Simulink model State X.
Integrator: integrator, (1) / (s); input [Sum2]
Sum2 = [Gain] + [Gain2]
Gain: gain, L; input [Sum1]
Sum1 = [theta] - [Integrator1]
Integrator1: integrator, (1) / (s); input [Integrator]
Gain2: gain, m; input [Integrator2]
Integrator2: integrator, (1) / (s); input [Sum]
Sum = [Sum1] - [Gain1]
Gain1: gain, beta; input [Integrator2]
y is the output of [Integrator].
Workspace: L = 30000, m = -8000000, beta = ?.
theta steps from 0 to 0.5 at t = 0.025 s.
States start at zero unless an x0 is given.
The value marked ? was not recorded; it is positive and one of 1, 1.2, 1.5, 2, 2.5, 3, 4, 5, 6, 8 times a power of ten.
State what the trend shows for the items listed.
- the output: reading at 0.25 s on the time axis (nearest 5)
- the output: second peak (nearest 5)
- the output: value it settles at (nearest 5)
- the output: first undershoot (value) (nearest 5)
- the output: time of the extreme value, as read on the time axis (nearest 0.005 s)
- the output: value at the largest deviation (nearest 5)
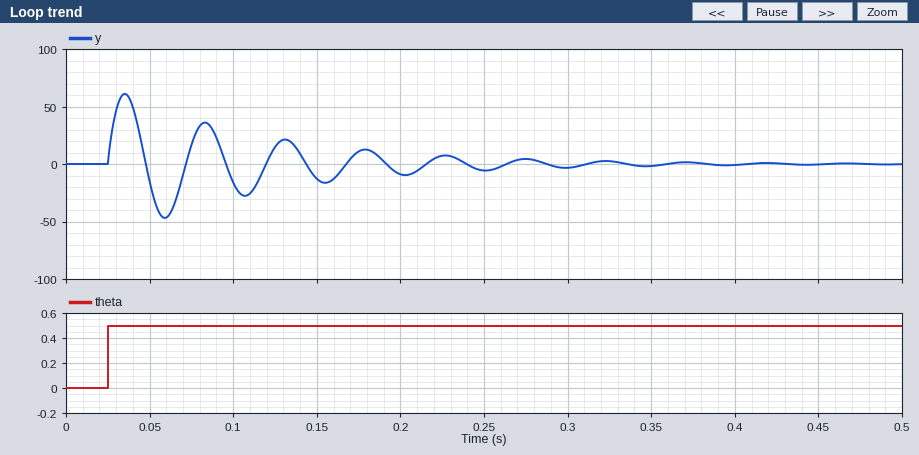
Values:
-5
35
0
-45
0.035 s
60
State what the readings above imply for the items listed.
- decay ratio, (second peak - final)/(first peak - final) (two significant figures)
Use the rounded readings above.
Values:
0.58
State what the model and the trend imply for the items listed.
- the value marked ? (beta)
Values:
600
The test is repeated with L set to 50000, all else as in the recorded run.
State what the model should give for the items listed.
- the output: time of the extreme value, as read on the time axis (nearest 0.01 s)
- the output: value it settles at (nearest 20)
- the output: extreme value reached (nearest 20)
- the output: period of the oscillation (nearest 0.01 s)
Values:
0.03 s
0
100
0.03 s
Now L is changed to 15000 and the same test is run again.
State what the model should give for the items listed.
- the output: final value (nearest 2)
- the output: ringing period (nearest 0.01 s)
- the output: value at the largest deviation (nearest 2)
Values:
0
0.16 s
18
